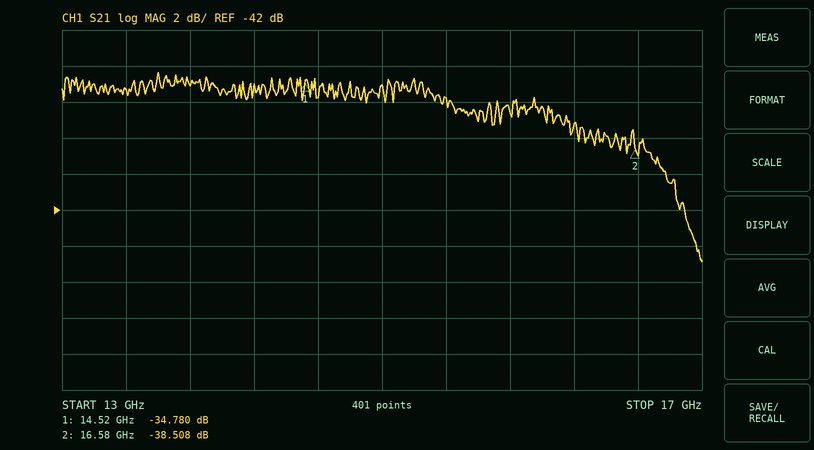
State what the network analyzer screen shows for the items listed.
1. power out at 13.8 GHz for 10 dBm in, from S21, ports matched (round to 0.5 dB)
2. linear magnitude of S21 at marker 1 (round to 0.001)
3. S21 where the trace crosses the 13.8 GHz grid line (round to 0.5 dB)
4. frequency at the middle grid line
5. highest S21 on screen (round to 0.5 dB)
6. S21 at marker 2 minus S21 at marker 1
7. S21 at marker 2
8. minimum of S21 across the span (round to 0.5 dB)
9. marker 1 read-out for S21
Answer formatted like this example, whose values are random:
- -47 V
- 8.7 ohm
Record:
- -25.0 dBm
- 0.018
- -35.0 dB
- 15 GHz
- -34.5 dB
- -3.728 dB
- -38.508 dB
- -45.0 dB
- -34.780 dB
